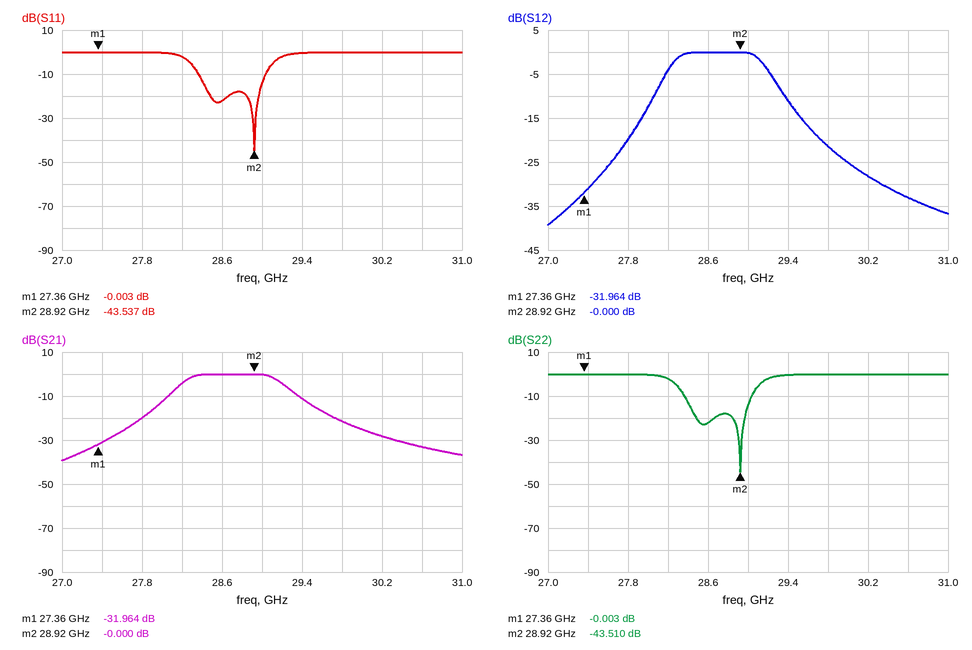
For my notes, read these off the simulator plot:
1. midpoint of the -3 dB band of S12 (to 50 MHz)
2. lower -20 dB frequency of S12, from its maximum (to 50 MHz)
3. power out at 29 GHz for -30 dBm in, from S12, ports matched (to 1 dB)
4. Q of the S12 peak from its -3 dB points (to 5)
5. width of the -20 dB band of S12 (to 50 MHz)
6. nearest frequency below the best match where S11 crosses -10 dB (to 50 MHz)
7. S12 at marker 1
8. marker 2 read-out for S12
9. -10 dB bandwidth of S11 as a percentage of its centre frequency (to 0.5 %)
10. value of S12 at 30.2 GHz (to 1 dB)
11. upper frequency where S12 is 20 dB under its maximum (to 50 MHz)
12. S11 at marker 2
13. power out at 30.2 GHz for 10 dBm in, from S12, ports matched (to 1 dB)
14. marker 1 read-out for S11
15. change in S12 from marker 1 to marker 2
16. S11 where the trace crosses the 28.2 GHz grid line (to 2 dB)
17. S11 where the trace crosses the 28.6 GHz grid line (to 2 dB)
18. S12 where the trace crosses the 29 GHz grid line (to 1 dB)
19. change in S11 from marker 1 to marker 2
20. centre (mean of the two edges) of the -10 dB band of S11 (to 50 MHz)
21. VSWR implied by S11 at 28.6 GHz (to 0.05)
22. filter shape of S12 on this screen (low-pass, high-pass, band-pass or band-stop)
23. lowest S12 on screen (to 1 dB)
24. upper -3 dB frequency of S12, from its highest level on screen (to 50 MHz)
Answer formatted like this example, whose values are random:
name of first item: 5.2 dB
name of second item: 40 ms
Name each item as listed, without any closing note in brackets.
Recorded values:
midpoint of the -3 dB band of S12: 28.70 GHz
lower -20 dB frequency of S12, from its maximum: 27.80 GHz
power out at 29 GHz for -30 dBm in, from S12, ports matched: -30 dBm
Q of the S12 peak from its -3 dB points: 30
width of the -20 dB band of S12: 1.95 GHz
nearest frequency below the best match where S11 crosses -10 dB: 28.35 GHz
S12 at marker 1: -31.964 dB
marker 2 read-out for S12: -0.000 dB
-10 dB bandwidth of S11 as a percentage of its centre frequency: 2.5 %
value of S12 at 30.2 GHz: -28 dB
upper frequency where S12 is 20 dB under its maximum: 29.75 GHz
S11 at marker 2: -43.537 dB
power out at 30.2 GHz for 10 dBm in, from S12, ports matched: -18 dBm
marker 1 read-out for S11: -0.003 dB
change in S12 from marker 1 to marker 2: 31.964 dB
S11 where the trace crosses the 28.2 GHz grid line: -2 dB
S11 where the trace crosses the 28.6 GHz grid line: -22 dB
S12 where the trace crosses the 29 GHz grid line: 0 dB
change in S11 from marker 1 to marker 2: -43.534 dB
centre (mean of the two edges) of the -10 dB band of S11: 28.70 GHz
VSWR implied by S11 at 28.6 GHz: 1.15
filter shape of S12 on this screen: band-pass
lowest S12 on screen: -39 dB
upper -3 dB frequency of S12, from its highest level on screen: 29.15 GHz
